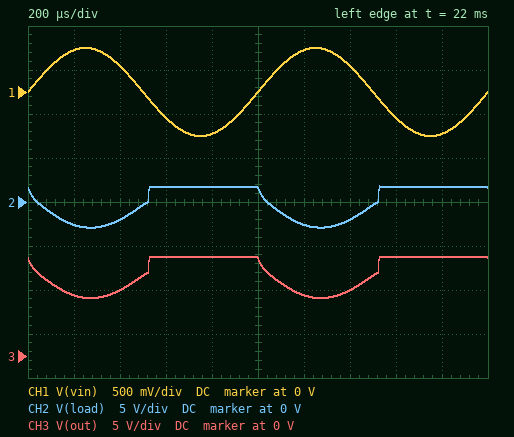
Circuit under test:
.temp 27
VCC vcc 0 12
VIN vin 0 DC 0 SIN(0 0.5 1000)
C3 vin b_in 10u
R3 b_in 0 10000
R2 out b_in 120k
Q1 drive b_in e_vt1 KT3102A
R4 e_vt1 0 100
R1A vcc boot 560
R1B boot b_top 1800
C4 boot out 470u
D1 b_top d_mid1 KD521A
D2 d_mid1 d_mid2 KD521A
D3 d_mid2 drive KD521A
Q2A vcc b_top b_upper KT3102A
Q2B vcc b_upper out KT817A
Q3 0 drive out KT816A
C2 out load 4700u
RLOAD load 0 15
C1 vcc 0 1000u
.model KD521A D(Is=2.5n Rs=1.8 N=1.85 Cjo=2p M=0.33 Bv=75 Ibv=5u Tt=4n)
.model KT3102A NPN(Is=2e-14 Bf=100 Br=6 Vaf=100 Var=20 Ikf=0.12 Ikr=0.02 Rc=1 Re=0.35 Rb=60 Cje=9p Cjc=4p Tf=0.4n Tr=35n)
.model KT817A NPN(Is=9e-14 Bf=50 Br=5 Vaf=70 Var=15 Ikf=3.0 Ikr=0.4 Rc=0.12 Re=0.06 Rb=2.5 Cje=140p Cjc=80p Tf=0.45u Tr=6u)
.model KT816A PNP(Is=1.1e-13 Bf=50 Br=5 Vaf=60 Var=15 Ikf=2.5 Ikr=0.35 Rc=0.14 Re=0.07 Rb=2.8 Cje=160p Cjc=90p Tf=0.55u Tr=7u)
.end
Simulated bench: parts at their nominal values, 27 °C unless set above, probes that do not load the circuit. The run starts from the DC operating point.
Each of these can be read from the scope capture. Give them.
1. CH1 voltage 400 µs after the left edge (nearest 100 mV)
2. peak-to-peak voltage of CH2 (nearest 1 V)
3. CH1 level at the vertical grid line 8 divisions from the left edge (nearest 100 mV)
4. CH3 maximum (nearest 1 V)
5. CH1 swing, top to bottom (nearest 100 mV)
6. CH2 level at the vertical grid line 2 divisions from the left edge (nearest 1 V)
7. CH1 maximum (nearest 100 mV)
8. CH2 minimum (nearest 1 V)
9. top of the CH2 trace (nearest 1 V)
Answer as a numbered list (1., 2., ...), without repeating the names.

1. 300 mV
2. 5 V
3. -300 mV
4. 11 V
5. 1.0 V
6. -2 V
7. 500 mV
8. -3 V
9. 2 V
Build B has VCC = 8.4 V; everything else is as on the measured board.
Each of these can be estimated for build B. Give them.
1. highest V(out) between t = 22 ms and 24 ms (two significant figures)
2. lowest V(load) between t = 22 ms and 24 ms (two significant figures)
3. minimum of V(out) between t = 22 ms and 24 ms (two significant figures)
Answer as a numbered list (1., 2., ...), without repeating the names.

1. 7.1 V
2. -2.3 V
3. 4.8 V
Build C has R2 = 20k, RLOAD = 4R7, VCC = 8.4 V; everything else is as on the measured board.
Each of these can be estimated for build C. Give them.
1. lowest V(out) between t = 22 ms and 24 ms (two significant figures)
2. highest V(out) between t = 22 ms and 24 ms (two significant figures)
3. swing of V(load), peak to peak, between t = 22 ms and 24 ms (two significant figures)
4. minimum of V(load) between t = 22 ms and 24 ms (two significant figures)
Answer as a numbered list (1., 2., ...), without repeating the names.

1. 2.8 V
2. 7.5 V
3. 4.7 V
4. -1.3 V
